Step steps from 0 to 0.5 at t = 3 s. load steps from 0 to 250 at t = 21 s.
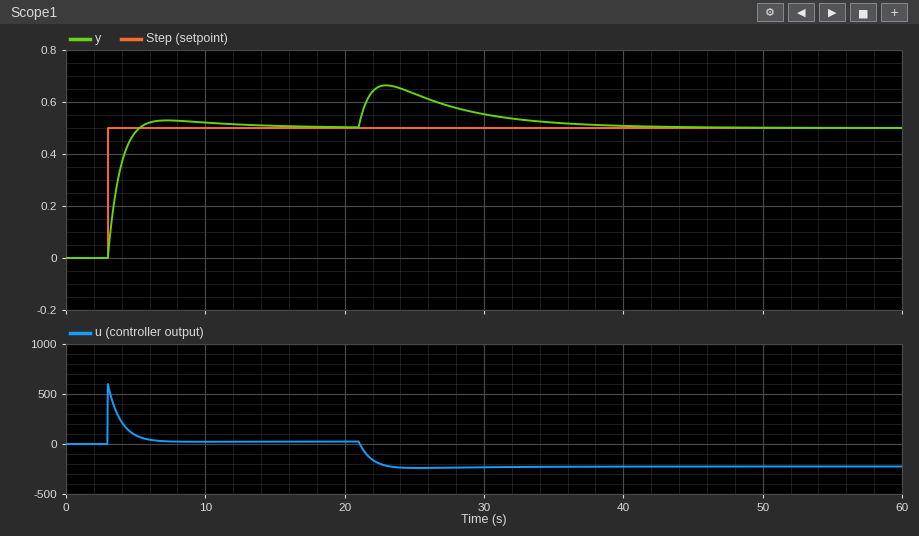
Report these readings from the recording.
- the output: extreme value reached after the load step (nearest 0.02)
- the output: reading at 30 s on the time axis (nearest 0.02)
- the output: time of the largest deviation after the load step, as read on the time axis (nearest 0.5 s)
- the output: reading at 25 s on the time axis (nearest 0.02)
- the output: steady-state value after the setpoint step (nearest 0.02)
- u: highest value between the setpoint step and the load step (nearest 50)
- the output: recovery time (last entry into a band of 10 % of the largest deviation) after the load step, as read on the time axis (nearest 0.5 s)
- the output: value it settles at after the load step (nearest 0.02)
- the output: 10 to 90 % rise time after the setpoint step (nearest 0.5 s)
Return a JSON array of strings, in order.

["0.66", "0.56", "23.0 s", "0.64", "0.50", "600", "36.5 s", "0.50", "1.5 s"]
